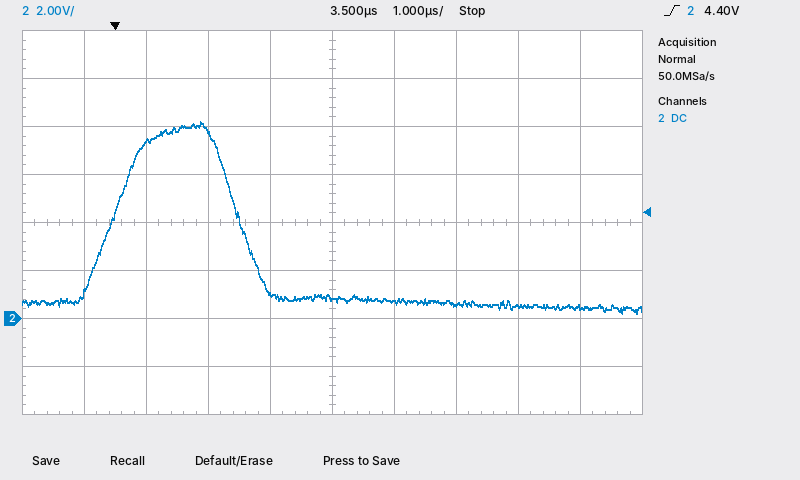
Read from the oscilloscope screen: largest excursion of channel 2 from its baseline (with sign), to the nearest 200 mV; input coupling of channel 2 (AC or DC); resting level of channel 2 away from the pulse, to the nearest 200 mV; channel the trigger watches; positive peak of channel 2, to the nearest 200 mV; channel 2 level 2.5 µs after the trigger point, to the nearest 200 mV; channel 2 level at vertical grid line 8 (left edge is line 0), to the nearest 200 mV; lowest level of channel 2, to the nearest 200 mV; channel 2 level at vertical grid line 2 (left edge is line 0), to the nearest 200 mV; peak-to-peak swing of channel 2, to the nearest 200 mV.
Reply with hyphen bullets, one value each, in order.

- +7.4 V
- DC
- 800 mV
- channel 2
- 8.2 V
- 1.0 V
- 600 mV
- 200 mV
- 7.4 V
- 8.0 V
